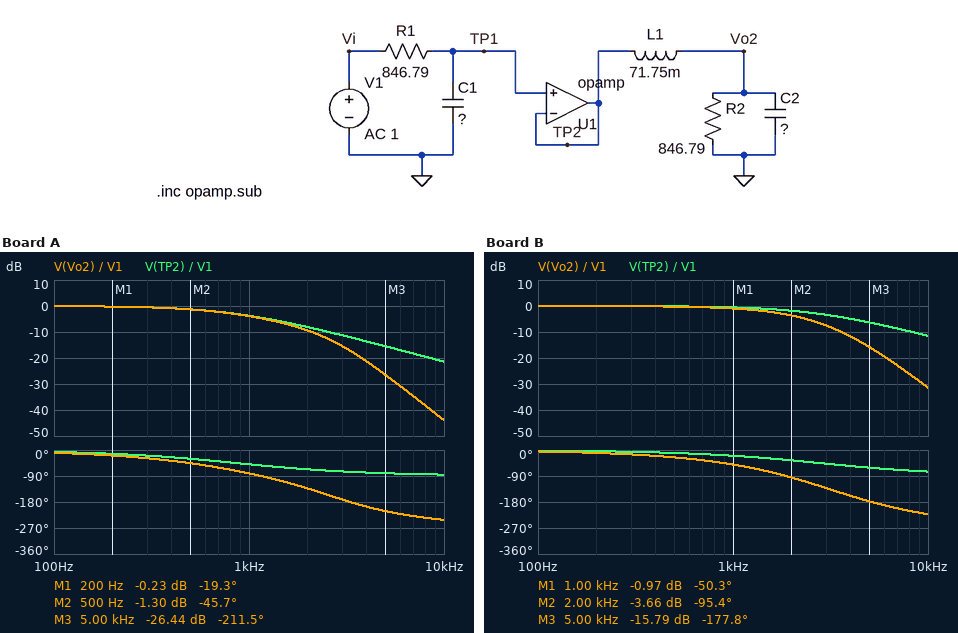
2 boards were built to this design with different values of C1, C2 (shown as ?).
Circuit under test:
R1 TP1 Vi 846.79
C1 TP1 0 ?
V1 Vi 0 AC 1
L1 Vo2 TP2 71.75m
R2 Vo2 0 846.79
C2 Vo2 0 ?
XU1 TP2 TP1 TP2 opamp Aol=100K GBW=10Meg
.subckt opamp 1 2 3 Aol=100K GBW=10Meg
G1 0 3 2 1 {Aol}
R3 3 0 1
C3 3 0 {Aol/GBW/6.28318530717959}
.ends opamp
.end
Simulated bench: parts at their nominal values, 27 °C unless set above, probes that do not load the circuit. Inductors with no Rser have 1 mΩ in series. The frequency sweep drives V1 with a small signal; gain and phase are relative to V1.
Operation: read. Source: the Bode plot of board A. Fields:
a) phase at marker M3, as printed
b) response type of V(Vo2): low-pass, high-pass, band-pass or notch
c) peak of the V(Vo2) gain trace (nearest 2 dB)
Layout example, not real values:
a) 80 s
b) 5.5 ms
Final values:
a) -211.5 deg
b) low-pass
c) 0 dB
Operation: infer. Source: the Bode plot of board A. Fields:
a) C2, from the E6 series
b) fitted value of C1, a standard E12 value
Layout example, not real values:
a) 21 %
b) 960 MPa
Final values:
a) 47 nF
b) 220 nF
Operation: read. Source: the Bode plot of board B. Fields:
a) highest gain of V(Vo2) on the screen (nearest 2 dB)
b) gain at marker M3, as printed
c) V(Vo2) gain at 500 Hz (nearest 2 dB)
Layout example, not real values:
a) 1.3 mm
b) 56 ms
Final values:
a) 0 dB
b) -15.79 dB
c) 0 dB
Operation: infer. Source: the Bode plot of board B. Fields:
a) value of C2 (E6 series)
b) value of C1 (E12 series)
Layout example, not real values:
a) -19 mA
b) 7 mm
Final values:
a) 33 nF
b) 68 nF
